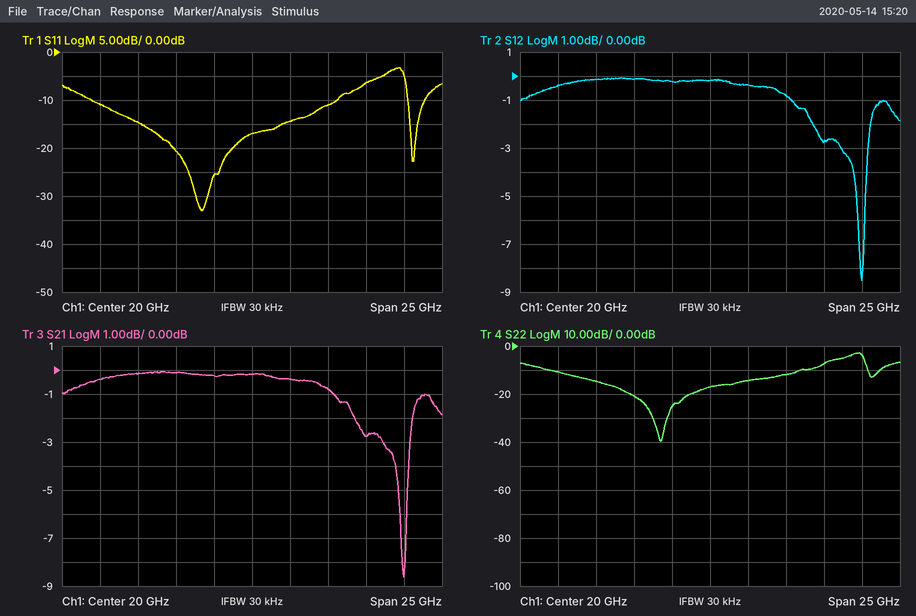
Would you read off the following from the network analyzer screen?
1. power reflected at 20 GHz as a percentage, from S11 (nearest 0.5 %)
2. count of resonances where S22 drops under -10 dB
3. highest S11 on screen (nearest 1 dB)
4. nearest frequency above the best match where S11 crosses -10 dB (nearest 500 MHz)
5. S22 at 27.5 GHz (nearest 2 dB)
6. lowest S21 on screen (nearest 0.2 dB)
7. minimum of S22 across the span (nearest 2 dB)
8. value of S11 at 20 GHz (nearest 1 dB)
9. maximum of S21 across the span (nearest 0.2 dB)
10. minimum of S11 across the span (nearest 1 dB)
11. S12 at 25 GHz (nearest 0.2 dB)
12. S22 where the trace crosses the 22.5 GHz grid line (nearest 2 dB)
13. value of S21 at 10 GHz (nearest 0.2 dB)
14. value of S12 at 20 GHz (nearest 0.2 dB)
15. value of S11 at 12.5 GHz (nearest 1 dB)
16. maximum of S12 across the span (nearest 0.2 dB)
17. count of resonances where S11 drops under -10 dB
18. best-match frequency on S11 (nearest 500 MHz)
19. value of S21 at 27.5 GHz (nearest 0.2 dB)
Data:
2.0 %
2
-3 dB
25.5 GHz
-8 dB
-8.6 dB
-40 dB
-17 dB
0.0 dB
-33 dB
-0.8 dB
-14 dB
-0.4 dB
-0.2 dB
-15 dB
0.0 dB
2
16.5 GHz
-2.8 dB
